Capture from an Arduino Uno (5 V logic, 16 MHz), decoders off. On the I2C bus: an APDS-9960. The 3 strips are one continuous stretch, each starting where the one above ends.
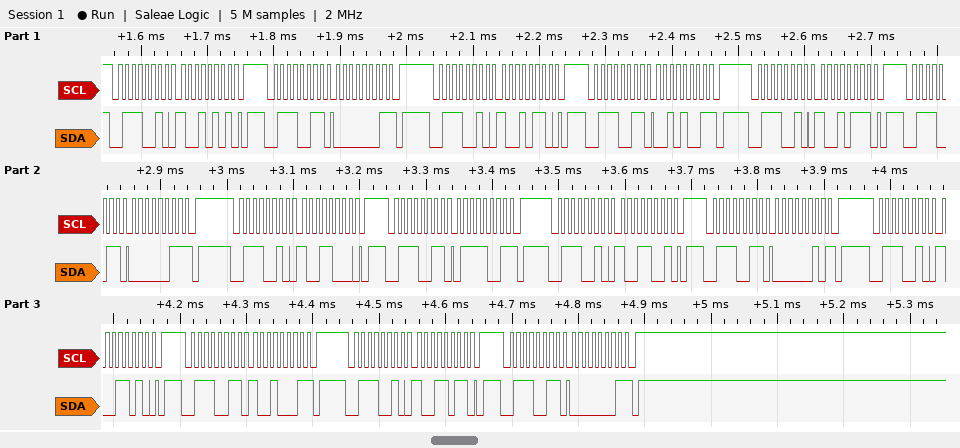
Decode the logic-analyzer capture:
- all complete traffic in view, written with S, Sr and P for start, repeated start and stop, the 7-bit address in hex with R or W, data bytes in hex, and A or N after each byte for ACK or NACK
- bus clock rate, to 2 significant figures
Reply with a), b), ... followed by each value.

a) S 39W A 95 A P S 39R A 01 N P S 39W A 96 A P S 39R A 29 N P S 39W A 97 A P S 39R A 03 N P S 39W A 98 A P S 39R A 79 N P S 39W A 99 A P S 39R A 02 N P S 39W A 9A A P S 39R A 91 N P S 39W A 9B A P S 39R A 01 N P
b) 100 kHz
